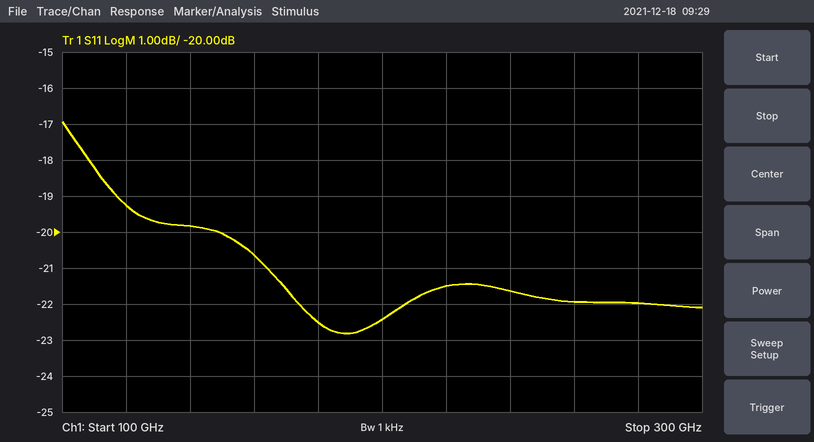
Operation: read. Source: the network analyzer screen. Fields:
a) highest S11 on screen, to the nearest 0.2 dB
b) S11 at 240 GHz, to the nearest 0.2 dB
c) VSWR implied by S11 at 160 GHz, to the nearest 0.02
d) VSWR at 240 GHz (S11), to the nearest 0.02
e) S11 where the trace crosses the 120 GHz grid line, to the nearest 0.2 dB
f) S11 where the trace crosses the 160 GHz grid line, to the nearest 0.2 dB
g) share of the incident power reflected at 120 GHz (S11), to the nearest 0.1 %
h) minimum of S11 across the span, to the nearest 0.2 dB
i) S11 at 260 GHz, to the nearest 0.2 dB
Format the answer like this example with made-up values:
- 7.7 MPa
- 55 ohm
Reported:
- -17.0 dB
- -21.6 dB
- 1.20
- 1.18
- -19.2 dB
- -20.6 dB
- 1.2 %
- -22.8 dB
- -22.0 dB
